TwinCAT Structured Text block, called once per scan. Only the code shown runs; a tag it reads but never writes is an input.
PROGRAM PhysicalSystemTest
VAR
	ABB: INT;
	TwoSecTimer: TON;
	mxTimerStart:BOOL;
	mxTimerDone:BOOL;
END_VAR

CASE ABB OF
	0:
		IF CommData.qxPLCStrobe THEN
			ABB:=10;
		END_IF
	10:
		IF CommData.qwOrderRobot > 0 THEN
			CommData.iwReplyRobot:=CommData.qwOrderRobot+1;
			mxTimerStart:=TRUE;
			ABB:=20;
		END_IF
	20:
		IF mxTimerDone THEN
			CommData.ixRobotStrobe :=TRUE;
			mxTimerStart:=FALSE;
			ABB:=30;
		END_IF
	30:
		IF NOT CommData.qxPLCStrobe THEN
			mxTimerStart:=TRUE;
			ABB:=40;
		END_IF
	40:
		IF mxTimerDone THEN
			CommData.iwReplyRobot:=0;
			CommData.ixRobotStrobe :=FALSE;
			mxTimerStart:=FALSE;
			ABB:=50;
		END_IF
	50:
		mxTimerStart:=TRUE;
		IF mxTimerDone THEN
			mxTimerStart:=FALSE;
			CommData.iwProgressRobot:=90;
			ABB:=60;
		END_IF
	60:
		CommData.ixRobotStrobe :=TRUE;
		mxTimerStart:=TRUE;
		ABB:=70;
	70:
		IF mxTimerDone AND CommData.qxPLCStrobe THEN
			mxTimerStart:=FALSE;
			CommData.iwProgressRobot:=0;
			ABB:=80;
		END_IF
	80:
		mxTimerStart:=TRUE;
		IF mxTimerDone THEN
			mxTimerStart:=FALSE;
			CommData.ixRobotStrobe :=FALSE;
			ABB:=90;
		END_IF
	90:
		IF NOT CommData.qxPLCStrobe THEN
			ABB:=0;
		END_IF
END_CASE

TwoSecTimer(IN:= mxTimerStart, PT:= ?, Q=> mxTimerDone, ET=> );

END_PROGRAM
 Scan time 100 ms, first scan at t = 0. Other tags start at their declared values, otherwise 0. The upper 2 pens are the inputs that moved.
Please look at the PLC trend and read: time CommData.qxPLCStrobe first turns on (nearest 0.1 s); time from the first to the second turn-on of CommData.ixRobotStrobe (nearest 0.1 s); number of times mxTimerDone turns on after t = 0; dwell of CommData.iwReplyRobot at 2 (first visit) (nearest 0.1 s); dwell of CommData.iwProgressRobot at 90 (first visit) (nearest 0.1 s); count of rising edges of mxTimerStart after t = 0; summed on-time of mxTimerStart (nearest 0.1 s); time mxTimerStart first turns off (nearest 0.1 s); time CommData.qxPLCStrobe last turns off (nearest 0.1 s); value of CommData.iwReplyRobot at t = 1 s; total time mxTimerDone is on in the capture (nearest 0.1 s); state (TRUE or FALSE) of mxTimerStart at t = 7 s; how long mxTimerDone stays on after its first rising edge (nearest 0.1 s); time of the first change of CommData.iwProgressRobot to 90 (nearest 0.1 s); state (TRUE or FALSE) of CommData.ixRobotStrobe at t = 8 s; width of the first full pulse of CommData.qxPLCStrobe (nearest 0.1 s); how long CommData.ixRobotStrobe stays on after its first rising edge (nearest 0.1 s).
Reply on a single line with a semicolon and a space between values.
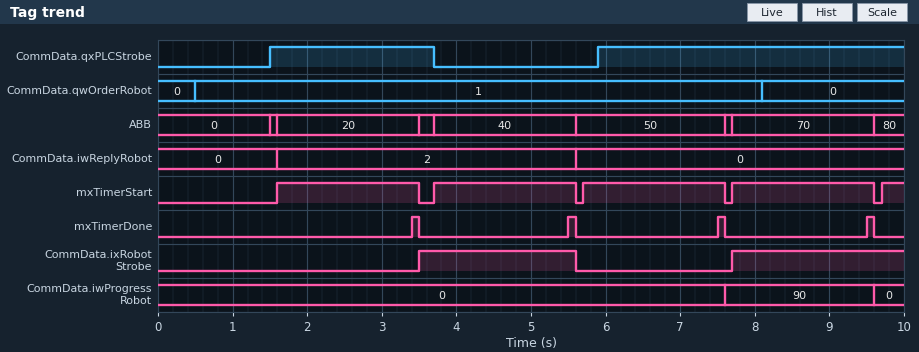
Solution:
1.5 s; 4.2 s; 4; 4.0 s; 2.0 s; 5; 7.9 s; 3.5 s; 3.7 s; 0; 0.4 s; TRUE; 0.1 s; 7.6 s; TRUE; 2.2 s; 2.1 s
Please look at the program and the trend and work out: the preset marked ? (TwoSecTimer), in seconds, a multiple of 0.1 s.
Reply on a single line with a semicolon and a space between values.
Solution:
1.8 s
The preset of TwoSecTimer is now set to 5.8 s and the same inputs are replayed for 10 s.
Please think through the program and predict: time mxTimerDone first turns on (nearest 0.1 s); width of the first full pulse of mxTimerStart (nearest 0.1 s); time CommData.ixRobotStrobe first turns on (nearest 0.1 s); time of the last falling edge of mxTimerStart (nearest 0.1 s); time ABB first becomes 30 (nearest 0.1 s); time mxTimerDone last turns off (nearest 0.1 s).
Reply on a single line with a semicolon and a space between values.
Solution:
7.4 s; 5.9 s; 7.5 s; 7.5 s; 7.5 s; 7.5 s
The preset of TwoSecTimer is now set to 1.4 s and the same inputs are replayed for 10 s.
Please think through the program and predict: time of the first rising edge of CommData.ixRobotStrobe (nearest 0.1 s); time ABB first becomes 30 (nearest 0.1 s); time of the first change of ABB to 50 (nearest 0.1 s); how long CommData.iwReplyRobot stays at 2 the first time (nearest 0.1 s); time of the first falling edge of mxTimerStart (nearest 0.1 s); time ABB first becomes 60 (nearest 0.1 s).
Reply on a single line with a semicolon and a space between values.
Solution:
3.1 s; 3.1 s; 5.2 s; 3.6 s; 3.1 s; 6.8 s
